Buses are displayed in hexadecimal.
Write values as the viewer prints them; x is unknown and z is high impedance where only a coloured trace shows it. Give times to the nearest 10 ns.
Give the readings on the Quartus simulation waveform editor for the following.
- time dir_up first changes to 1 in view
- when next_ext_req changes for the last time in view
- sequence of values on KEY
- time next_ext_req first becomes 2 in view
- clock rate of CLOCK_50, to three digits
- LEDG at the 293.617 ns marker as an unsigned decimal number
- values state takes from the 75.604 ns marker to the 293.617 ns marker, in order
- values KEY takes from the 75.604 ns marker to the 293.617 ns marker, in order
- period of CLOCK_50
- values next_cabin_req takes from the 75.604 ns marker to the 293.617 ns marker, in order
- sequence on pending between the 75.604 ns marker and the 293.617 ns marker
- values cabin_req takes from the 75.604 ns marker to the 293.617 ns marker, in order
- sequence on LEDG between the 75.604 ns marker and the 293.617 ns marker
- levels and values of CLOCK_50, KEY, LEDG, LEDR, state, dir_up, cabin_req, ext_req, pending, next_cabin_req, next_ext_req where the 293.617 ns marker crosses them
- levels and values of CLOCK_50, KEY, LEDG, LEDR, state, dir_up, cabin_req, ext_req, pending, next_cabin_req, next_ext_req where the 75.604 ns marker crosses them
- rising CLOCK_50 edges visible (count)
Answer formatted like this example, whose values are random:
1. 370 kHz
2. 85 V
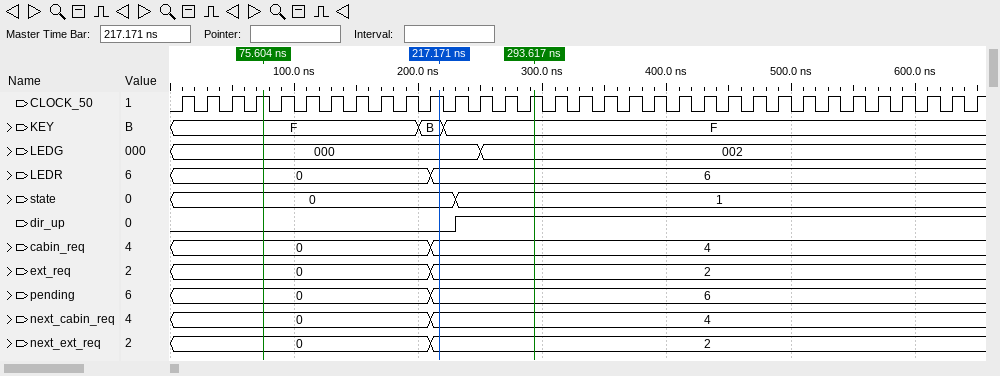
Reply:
1. 230 ns
2. 210 ns
3. F, B, F
4. 210 ns
5. 50.0 MHz
6. 2
7. 0, 1
8. F, B, F
9. 20 ns
10. 0, 4
11. 0, 6
12. 0, 4
13. 000, 002
14. CLOCK_50=1, KEY=F, LEDG=002, LEDR=6, state=1, dir_up=1, cabin_req=4, ext_req=2, pending=6, next_cabin_req=4, next_ext_req=2
15. CLOCK_50=1, KEY=F, LEDG=000, LEDR=0, state=0, dir_up=0, cabin_req=0, ext_req=0, pending=0, next_cabin_req=0, next_ext_req=0
16. 33
